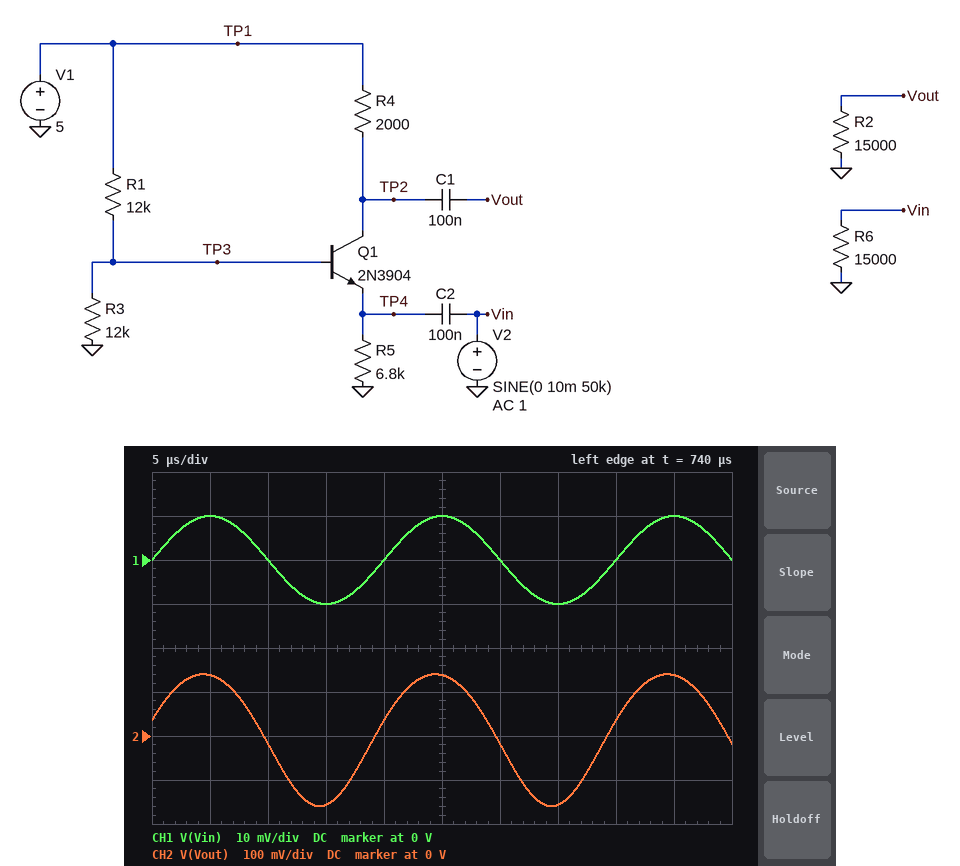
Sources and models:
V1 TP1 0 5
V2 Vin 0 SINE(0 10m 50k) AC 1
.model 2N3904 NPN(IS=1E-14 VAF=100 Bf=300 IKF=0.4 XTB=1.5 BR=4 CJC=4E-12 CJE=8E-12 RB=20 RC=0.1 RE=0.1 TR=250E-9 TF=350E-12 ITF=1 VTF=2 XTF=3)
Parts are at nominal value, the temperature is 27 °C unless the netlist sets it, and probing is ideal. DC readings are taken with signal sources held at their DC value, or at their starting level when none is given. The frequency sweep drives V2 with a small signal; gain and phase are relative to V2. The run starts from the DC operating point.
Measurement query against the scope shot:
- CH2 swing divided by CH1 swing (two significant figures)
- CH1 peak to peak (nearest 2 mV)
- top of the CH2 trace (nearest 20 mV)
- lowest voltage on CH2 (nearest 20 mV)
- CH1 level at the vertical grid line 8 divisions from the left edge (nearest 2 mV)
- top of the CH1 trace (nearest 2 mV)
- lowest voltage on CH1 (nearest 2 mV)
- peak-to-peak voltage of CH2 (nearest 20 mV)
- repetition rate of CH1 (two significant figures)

15
20 mV
140 mV
-160 mV
0 V
10 mV
-10 mV
300 mV
50 kHz
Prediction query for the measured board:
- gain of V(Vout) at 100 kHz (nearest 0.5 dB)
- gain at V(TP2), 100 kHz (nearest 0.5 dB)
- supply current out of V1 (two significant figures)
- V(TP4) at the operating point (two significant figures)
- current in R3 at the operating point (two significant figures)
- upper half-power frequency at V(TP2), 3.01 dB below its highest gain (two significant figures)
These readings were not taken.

23.5 dB
23.5 dB
480 µA
1.9 V
210 µA
490 kHz
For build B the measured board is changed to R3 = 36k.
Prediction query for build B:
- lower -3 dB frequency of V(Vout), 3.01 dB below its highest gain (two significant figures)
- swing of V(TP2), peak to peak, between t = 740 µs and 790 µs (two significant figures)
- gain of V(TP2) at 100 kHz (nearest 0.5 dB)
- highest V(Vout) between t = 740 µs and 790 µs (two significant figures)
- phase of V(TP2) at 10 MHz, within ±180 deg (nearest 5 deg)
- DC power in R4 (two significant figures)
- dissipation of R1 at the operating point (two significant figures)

17 kHz
390 mV
25.5 dB
190 mV
-25 deg
410 µW
130 µW
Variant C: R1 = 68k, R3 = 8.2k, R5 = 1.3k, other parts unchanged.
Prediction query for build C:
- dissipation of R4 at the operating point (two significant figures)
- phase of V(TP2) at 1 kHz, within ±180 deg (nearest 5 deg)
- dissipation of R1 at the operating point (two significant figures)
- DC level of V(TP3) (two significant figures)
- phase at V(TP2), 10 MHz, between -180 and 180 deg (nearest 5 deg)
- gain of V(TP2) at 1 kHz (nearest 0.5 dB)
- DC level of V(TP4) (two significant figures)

120 nW
60 deg
290 µW
540 mV
55 deg
-11.5 dB
10 mV
